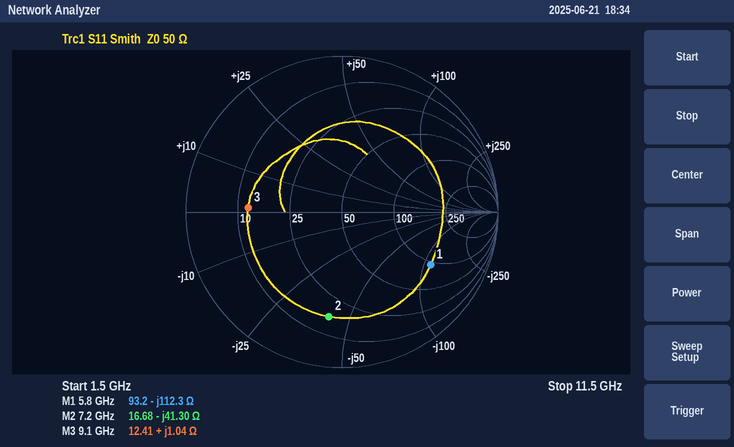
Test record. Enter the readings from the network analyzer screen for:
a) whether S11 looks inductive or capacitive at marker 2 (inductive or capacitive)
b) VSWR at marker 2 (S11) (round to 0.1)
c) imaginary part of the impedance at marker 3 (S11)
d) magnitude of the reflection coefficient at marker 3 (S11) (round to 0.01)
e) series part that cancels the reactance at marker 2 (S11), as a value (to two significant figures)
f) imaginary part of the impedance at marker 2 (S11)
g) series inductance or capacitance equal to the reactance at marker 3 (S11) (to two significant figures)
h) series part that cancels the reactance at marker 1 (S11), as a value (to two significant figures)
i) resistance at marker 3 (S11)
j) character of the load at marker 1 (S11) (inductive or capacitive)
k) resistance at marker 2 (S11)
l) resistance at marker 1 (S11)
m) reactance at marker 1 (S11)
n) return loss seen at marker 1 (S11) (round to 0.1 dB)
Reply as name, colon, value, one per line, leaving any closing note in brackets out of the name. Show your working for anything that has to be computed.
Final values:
whether S11 looks inductive or capacitive at marker 2: capacitive
VSWR at marker 2 (S11): 5.2
imaginary part of the impedance at marker 3: +1.04 Ω
magnitude of the reflection coefficient at marker 3 (S11): 0.60
series part that cancels the reactance at marker 2 (S11), as a value: L = 41.3 Ω/(2π × 7.2 GHz) ≈ 913 pH, so 910 pH to two significant figures
imaginary part of the impedance at marker 2: -41.30 Ω
series inductance or capacitance equal to the reactance at marker 3 (S11): L = 1.04 Ω/(2π × 9.1 GHz) ≈ 18 pH
series part that cancels the reactance at marker 1 (S11), as a value: L = 112.3 Ω/(2π × 5.8 GHz) ≈ 3.1 nH
resistance at marker 3: 12.41 Ω
character of the load at marker 1 (S11): capacitive
resistance at marker 2: 16.68 Ω
resistance at marker 1: 93.2 Ω
reactance at marker 1: -112.3 Ω
return loss seen at marker 1 (S11): 3.6 dB
